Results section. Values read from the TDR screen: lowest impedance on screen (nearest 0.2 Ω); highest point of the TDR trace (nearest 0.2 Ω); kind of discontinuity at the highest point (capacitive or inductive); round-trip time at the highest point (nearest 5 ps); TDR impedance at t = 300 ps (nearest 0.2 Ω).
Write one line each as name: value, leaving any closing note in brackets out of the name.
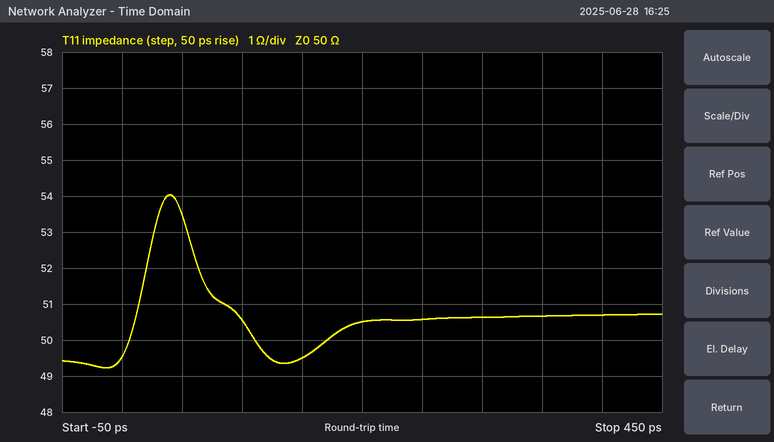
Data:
lowest impedance on screen: 49.2 Ω
highest point of the TDR trace: 54.0 Ω
kind of discontinuity at the highest point: inductive
round-trip time at the highest point: 40 ps
TDR impedance at t = 300 ps: 50.6 Ω
